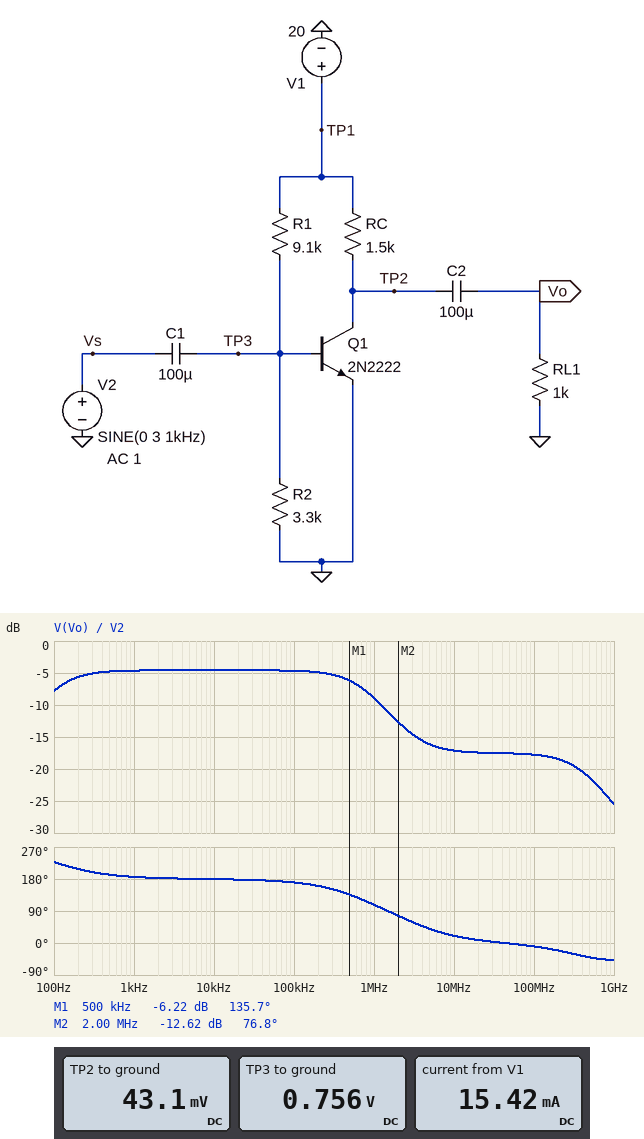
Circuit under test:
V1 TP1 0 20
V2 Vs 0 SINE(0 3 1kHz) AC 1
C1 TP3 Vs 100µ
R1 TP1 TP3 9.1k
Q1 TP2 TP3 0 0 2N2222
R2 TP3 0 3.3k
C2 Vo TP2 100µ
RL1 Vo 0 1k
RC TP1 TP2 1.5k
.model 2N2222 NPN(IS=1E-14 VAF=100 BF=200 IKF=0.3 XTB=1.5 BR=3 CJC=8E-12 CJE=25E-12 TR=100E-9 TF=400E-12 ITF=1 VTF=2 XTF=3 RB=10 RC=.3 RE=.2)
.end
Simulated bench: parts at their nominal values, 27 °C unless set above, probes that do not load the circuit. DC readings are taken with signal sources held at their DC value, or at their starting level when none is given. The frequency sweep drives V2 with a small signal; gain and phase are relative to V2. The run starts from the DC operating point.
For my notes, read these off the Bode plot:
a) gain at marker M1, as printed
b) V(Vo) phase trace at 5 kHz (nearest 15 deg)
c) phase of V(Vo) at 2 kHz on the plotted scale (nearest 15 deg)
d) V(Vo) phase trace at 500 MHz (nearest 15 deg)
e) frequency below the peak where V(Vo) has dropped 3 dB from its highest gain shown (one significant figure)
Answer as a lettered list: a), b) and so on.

a) -6.22 dB
b) 180 deg
c) 180 deg
d) -45 deg
e) 100 Hz
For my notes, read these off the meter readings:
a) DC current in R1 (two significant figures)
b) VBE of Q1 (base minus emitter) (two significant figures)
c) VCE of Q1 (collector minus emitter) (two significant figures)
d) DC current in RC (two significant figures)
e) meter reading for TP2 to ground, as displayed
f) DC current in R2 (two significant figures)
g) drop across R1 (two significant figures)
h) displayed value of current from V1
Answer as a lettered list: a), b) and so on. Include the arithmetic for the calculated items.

a) (20 V - 756 mV) / 9.1 kΩ = 2.1 mA
b) 756 mV = 760 mV
c) 43.1 mV = 43 mV
d) (20 V - 43.1 mV) / 1.5 kΩ = 13 mA
e) 43.1 mV
f) (756 mV) / 3.3 kΩ = 230 µA
g) 20 V - 756 mV = 19 V
h) 15.42 mA
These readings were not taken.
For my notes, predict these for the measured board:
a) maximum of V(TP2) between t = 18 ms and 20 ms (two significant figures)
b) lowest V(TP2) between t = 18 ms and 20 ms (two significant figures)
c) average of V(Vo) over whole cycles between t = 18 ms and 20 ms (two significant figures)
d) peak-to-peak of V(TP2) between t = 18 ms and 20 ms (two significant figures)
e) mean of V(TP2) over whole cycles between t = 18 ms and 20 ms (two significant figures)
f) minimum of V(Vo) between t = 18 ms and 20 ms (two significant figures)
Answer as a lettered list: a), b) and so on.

a) 8.7 V
b) 25 mV
c) 6.0 V
d) 8.7 V
e) 7.1 V
f) -1.1 V
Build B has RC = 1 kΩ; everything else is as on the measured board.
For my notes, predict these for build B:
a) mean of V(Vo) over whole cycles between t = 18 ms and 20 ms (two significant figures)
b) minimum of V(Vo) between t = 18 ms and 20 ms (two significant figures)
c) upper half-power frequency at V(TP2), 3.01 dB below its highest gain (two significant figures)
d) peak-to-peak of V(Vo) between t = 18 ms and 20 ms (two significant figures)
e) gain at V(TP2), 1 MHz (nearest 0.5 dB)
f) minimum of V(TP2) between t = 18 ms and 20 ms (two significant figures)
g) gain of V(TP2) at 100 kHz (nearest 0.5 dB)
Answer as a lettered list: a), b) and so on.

a) 7.4 V
b) -1.4 V
c) 690 kHz
d) 11 V
e) -7.5 dB
f) 31 mV
g) -2.5 dB
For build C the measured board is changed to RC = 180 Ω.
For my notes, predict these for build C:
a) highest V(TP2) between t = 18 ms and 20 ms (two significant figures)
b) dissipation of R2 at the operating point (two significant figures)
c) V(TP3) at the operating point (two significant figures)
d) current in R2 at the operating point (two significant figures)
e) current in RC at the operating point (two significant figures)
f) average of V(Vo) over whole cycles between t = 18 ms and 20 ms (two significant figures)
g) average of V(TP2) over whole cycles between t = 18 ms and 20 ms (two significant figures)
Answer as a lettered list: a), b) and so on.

a) 17 V
b) 210 µW
c) 830 mV
d) 250 µA
e) 110 mA
f) 12 V
g) 14 V
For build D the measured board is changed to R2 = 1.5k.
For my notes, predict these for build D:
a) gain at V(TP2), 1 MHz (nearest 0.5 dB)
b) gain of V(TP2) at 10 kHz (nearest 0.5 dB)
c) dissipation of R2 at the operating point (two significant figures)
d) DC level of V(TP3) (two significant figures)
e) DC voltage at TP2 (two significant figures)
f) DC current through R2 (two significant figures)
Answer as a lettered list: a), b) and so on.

a) -7.0 dB
b) -3.0 dB
c) 380 µW
d) 750 mV
e) 46 mV
f) 500 µA
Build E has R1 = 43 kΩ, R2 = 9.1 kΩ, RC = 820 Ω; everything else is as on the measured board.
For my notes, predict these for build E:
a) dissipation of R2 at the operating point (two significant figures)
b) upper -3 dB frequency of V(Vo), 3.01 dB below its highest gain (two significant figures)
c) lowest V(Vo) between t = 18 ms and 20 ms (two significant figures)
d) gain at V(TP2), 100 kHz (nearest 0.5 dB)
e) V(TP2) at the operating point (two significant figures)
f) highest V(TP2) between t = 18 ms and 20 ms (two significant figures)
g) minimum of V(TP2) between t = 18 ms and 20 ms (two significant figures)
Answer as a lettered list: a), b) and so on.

a) 62 µW
b) 690 kHz
c) -1.6 V
d) 17.0 dB
e) 110 mV
f) 12 V
g) 35 mV
